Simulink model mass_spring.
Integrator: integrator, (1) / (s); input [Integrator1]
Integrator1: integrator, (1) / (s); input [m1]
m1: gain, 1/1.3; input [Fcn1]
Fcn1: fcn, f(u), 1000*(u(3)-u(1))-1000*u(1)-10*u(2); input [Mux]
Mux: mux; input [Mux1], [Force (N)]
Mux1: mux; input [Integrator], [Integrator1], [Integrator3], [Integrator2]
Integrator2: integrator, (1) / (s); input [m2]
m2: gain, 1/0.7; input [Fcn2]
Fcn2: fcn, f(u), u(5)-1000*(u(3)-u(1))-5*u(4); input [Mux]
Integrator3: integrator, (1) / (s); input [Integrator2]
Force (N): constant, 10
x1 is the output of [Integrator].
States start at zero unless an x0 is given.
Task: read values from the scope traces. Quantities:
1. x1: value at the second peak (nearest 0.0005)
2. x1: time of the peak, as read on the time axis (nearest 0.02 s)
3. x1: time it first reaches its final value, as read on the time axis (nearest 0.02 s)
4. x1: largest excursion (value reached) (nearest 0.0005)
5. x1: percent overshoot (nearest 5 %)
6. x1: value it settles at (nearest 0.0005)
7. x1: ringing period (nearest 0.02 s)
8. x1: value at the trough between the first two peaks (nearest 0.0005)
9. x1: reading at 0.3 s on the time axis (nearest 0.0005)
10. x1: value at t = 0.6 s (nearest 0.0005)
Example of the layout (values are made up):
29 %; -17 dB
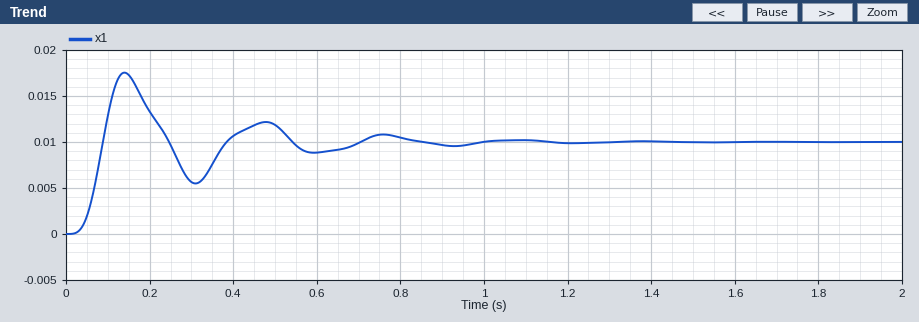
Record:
0.0120; 0.14 s; 0.08 s; 0.0175; 75 %; 0.0100; 0.34 s; 0.0055; 0.0055; 0.0090
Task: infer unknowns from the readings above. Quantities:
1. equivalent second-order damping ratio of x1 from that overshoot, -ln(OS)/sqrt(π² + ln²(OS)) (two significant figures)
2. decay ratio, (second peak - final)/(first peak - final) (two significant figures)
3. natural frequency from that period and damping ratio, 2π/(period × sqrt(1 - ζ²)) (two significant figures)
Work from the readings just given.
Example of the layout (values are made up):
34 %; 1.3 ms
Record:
0.091; 0.27; 19 rad/s
